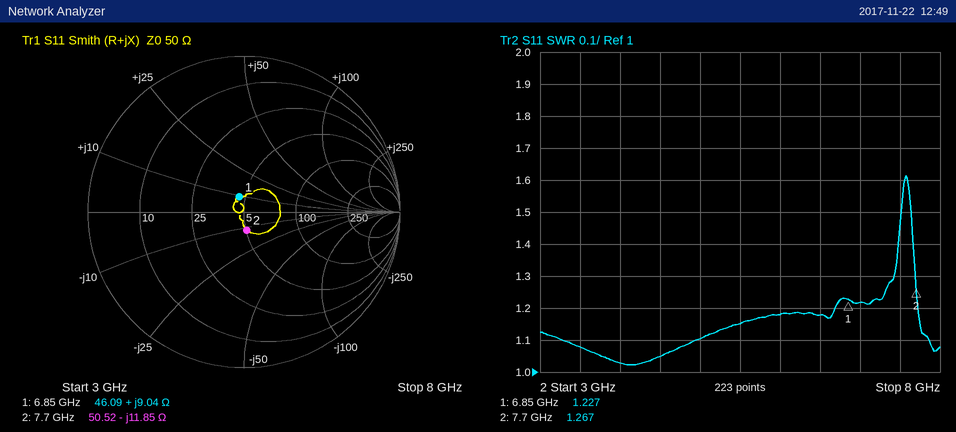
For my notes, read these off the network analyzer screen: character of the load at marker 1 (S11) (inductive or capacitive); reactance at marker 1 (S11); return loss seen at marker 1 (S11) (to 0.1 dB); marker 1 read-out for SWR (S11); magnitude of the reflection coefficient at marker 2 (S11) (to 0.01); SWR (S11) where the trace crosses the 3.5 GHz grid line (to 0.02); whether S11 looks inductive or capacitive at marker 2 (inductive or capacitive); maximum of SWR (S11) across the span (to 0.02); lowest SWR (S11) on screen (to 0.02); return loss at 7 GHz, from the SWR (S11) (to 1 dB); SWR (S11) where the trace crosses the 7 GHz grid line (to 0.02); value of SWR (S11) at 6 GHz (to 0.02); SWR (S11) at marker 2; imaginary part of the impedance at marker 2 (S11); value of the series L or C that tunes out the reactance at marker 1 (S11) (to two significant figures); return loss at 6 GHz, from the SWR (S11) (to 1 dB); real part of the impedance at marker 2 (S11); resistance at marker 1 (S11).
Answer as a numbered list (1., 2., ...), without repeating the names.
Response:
1. inductive
2. +9.04 Ω
3. 19.8 dB
4. 1.227
5. 0.12
6. 1.08
7. capacitive
8. 1.62
9. 1.02
10. 20 dB
11. 1.22
12. 1.18
13. 1.267
14. -11.85 Ω
15. 2.6 pF
16. 22 dB
17. 50.52 Ω
18. 46.09 Ω
